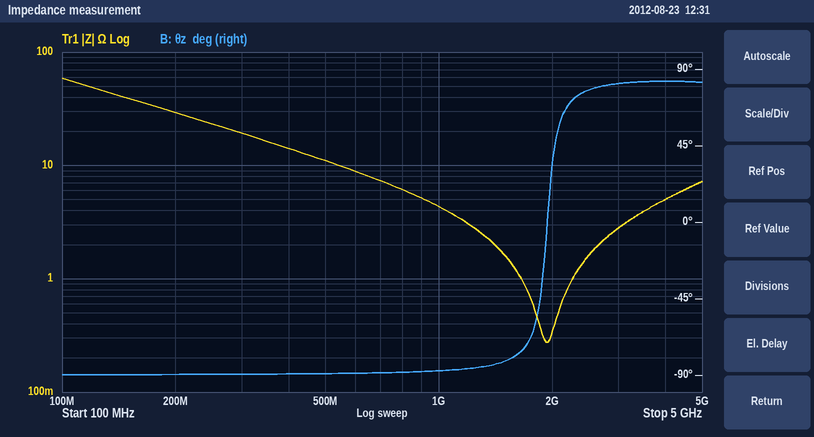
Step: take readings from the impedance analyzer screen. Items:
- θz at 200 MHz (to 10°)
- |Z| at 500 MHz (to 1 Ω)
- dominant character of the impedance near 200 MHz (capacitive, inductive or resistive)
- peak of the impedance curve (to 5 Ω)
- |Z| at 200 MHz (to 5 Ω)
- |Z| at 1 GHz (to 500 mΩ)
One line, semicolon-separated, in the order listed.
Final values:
-90°; 11 Ω; capacitive; 60 Ω; 30 Ω; 4.5 Ω
